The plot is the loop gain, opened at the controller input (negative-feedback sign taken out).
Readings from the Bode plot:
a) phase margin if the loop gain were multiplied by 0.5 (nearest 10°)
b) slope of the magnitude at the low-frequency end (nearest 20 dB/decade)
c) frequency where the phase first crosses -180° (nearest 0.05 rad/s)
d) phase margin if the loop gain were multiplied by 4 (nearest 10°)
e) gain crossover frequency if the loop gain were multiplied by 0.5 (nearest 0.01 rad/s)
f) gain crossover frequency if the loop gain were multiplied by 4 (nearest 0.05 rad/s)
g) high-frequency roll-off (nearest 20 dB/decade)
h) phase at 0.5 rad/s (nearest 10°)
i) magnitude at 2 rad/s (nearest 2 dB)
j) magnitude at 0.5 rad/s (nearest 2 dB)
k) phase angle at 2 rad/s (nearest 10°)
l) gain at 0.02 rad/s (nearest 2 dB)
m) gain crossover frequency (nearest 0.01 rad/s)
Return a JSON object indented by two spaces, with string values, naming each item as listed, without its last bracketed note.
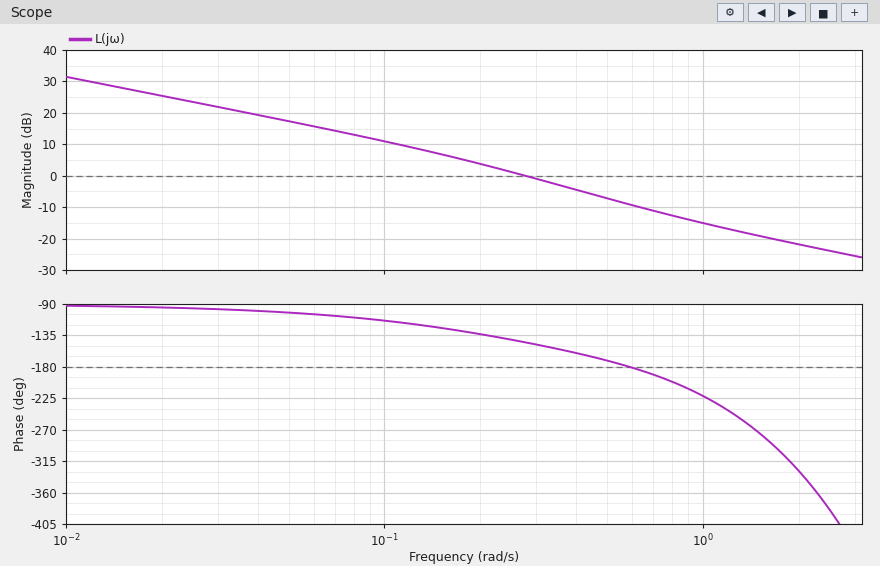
{
  "phase margin if the loop gain were multiplied by 0.5": "50°",
  "slope of the magnitude at the low-frequency end": "-20 dB/decade",
  "frequency where the phase first crosses -180°": "0.60 rad/s",
  "phase margin if the loop gain were multiplied by 4": "-20°",
  "gain crossover frequency if the loop gain were multiplied by 0.5": "0.16 rad/s",
  "gain crossover frequency if the loop gain were multiplied by 4": "0.75 rad/s",
  "high-frequency roll-off": "-20 dB/decade",
  "phase at 0.5 rad/s": "-170°",
  "magnitude at 2 rad/s": "-22 dB",
  "magnitude at 0.5 rad/s": "-8 dB",
  "phase angle at 2 rad/s": "-330°",
  "gain at 0.02 rad/s": "26 dB",
  "gain crossover frequency": "0.28 rad/s"
}
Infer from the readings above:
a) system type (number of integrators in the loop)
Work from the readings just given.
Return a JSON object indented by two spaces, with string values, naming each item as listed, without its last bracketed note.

{
  "system type": "1"
}
